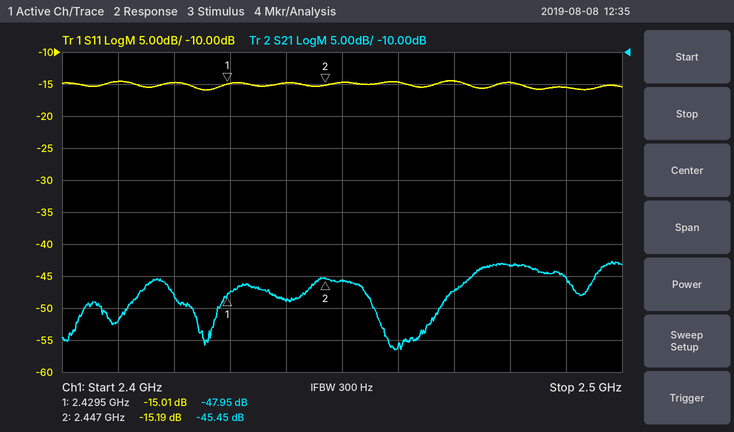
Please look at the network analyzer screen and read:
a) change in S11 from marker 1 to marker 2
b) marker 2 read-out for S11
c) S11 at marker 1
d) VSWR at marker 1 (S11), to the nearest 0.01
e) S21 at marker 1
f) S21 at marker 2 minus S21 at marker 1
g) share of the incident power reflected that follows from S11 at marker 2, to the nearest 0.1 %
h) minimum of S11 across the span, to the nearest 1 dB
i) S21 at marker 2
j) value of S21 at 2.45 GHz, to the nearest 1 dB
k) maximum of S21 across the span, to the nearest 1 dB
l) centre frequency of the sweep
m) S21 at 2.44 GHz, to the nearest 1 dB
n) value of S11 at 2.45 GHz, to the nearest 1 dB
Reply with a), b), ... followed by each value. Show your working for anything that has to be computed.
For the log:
a) -15.19 − (-15.01) = -0.18 dB
b) -15.19 dB
c) -15.01 dB
d) (1 + 0.1776)/(1 − 0.1776) ≈ 1.43
e) -47.95 dB
f) -45.45 − (-47.95) = 2.50 dB
g) 10^(-15.19/10) ≈ 3.0 %
h) -16 dB
i) -45.45 dB
j) -46 dB
k) -43 dB
l) 2.45 GHz
m) -49 dB
n) -15 dB
